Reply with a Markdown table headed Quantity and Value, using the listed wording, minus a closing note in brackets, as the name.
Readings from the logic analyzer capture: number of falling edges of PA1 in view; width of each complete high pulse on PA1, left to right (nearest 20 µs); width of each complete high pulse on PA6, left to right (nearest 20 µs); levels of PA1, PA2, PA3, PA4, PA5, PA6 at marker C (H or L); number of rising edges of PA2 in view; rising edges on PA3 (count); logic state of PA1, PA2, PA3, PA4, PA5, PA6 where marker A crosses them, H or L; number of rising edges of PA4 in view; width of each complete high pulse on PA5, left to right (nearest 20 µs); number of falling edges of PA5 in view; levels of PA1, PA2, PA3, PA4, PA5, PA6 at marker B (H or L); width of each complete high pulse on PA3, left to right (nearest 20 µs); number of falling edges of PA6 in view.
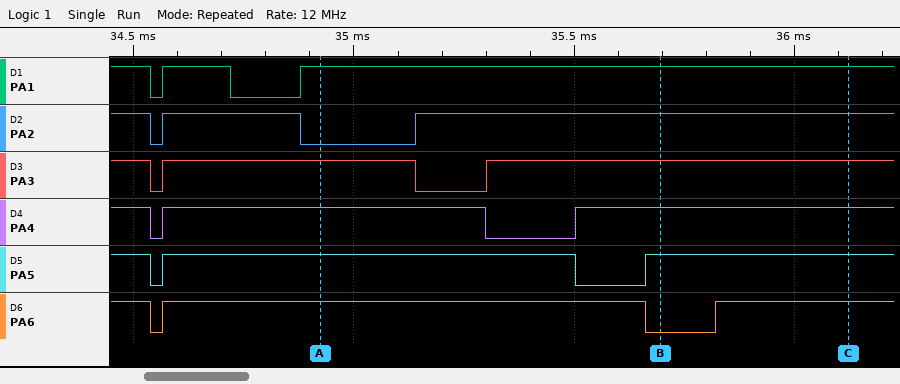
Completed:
| Quantity | Value |
|---|---|
| number of falling edges of PA1 in view | 2 |
| width of each complete high pulse on PA1, left to right | 160 µs |
| width of each complete high pulse on PA6, left to right | 1100 µs |
| levels of PA1, PA2, PA3, PA4, PA5, PA6 at marker C | PA1=H, PA2=H, PA3=H, PA4=H, PA5=H, PA6=H |
| number of rising edges of PA2 in view | 2 |
| rising edges on PA3 | 2 |
| logic state of PA1, PA2, PA3, PA4, PA5, PA6 where marker A crosses them, H or L | PA1=H, PA2=L, PA3=H, PA4=H, PA5=H, PA6=H |
| number of rising edges of PA4 in view | 2 |
| width of each complete high pulse on PA5, left to right | 940 µs |
| number of falling edges of PA5 in view | 2 |
| levels of PA1, PA2, PA3, PA4, PA5, PA6 at marker B | PA1=H, PA2=H, PA3=H, PA4=H, PA5=H, PA6=L |
| width of each complete high pulse on PA3, left to right | 580 µs |
| number of falling edges of PA6 in view | 2 |
